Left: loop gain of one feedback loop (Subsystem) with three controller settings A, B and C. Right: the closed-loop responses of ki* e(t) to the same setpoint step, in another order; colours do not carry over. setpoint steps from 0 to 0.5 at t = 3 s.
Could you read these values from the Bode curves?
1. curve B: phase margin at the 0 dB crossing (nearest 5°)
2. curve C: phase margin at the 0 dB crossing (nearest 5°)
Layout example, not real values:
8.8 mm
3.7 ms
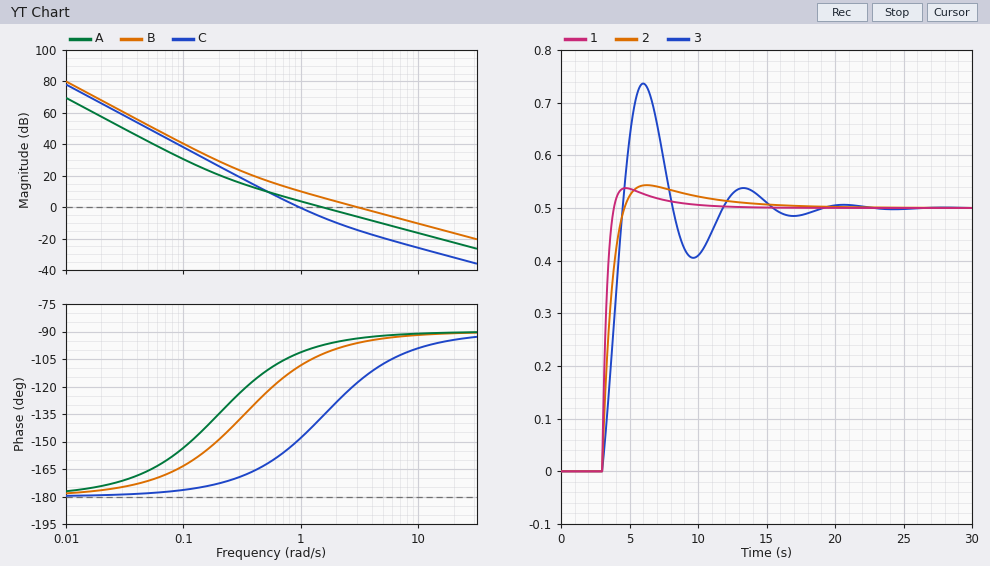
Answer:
85°
30°
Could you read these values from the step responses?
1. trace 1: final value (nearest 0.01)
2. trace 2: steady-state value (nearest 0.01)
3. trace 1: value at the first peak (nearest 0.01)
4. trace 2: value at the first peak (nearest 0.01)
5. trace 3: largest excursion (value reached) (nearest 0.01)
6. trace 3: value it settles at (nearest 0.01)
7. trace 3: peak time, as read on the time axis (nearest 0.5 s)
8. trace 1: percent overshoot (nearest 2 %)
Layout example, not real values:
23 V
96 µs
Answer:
0.50
0.50
0.54
0.54
0.74
0.50
6.0 s
8 %
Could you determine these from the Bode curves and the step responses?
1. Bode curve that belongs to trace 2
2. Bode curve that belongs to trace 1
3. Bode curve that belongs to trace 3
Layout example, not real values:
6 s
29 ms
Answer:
A
B
C
